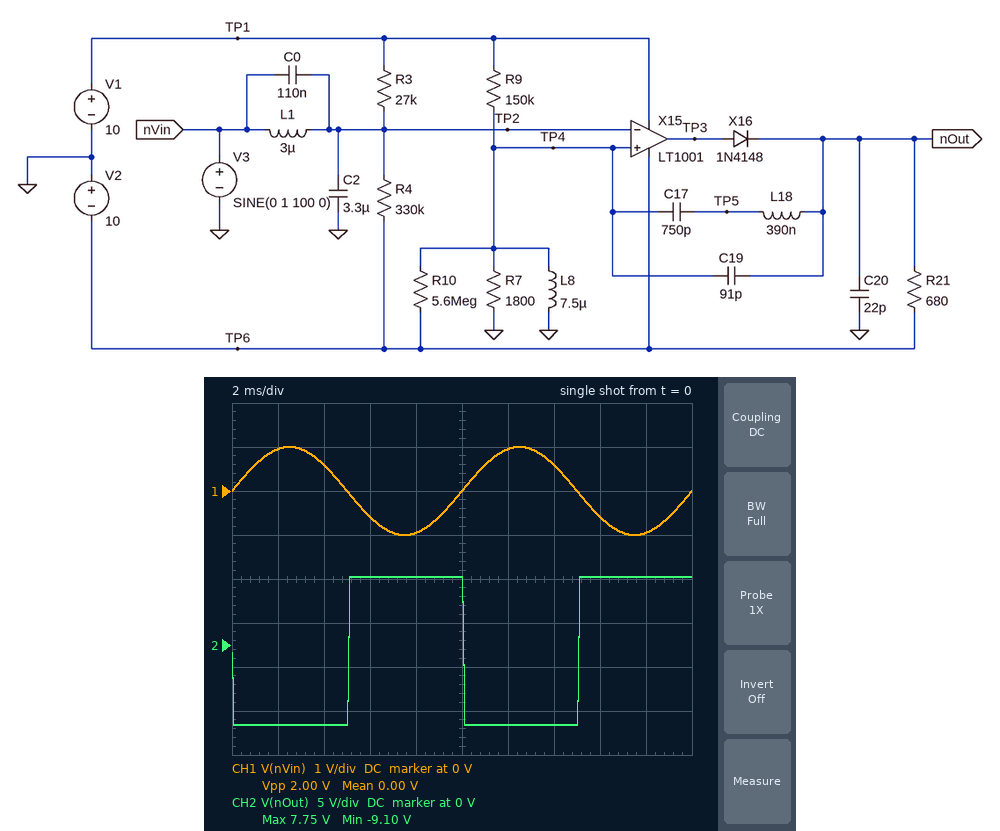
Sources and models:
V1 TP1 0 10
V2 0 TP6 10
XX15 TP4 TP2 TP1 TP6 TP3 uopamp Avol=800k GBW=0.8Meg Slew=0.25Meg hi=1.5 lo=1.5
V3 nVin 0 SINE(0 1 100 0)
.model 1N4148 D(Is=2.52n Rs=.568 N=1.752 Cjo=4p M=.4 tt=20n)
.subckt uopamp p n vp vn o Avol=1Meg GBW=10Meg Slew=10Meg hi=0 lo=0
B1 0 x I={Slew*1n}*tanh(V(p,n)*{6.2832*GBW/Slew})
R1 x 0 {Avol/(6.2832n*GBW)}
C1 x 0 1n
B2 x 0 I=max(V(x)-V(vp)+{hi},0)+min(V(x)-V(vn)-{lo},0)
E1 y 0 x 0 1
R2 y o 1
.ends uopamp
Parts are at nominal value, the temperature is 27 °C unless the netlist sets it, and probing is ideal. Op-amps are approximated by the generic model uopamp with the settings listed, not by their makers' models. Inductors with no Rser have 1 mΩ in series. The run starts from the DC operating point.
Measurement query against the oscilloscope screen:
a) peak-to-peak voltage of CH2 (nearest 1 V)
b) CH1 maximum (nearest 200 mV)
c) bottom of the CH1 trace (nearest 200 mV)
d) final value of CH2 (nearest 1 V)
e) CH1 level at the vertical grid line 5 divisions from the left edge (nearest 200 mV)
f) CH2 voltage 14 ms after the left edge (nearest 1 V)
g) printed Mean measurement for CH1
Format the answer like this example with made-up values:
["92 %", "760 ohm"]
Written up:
["17 V", "1.0 V", "-1.0 V", "8 V", "0 V", "-9 V", "0.00 V"]
